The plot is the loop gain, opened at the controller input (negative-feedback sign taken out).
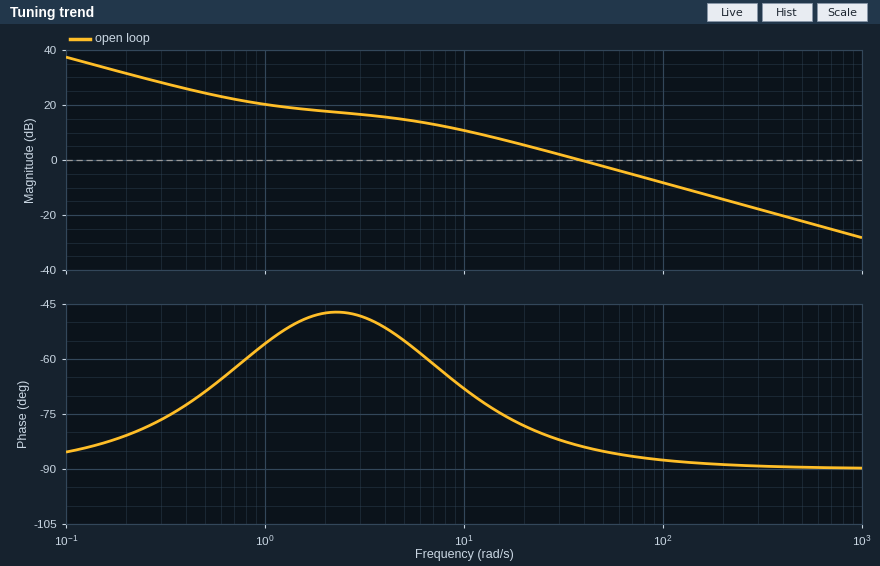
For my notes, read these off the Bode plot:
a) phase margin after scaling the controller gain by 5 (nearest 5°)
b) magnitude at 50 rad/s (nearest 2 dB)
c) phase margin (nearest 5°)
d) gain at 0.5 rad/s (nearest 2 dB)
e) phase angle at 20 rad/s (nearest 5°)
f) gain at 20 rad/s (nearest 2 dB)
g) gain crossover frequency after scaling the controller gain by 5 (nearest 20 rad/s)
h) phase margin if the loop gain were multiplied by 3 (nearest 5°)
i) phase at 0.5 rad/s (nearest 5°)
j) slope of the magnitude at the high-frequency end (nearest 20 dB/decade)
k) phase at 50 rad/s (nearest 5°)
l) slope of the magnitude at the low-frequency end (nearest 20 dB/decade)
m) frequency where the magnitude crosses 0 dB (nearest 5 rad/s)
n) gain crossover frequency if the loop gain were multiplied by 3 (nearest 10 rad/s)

90°
-2 dB
95°
24 dB
-80°
6 dB
200 rad/s
90°
-70°
-20 dB/decade
-85°
-20 dB/decade
40 rad/s
120 rad/s
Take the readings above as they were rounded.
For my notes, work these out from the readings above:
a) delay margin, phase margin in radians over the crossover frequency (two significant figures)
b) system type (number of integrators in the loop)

0.041 s
1
